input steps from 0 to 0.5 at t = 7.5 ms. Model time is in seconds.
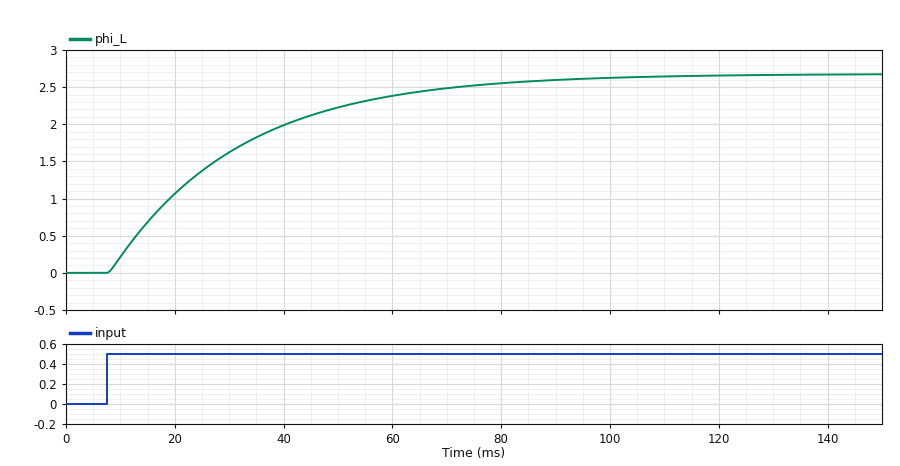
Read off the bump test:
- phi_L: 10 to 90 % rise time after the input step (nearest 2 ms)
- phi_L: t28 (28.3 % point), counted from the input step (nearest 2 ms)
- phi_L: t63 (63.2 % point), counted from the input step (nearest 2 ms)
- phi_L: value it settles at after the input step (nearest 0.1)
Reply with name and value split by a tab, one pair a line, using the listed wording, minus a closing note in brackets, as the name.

phi_L: 10 to 90 % rise time after the input step	52 ms
phi_L: t28 (28.3 % point), counted from the input step	8 ms
phi_L: t63 (63.2 % point), counted from the input step	24 ms
phi_L: value it settles at after the input step	2.7
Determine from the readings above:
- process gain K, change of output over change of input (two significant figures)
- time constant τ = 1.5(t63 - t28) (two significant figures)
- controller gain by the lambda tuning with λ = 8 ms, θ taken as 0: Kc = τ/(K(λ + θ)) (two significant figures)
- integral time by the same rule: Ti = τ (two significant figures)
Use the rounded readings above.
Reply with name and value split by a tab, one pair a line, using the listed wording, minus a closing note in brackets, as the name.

process gain K, change of output over change of input	5.4
time constant τ = 1.5(t63 - t28)	24 ms
controller gain by the lambda tuning with λ = 8 ms, θ taken as 0: Kc = τ/(K(λ + θ))	0.56
integral time by the same rule: Ti = τ	24 ms
